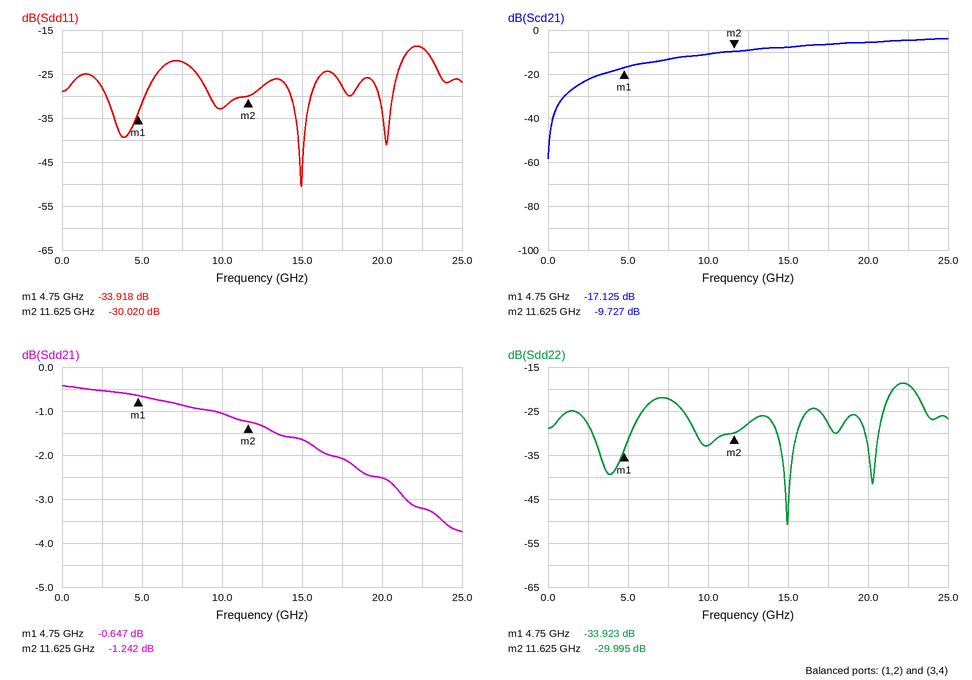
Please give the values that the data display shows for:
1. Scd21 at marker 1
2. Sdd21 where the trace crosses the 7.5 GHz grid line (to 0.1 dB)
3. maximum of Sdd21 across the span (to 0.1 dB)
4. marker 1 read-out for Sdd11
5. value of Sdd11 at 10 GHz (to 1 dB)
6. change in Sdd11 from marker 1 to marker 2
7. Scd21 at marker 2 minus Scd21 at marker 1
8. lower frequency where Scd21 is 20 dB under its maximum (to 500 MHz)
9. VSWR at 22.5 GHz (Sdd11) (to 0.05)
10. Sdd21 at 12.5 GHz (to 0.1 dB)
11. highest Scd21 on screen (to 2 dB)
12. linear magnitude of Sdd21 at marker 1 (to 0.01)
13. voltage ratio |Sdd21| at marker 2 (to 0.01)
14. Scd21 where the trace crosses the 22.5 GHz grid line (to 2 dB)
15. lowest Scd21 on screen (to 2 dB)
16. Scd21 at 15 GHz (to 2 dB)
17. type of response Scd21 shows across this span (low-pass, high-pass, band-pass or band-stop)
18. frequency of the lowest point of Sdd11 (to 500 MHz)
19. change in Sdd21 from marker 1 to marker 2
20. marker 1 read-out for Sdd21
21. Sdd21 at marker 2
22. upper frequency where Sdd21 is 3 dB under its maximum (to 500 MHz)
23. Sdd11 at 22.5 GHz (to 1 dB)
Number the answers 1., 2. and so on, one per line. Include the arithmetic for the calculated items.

1. -17.125 dB
2. -0.9 dB
3. -0.4 dB
4. -33.918 dB
5. -33 dB
6. -30.02 − (-33.918) = 3.898 dB
7. -9.727 − (-17.125) = 7.398 dB
8. 2.0 GHz
9. |Γ| = 10^(-19/20) = 0.1122; VSWR = (1 + 0.1122)/(1 − 0.1122) ≈ 1.25
10. -1.3 dB
11. -4 dB
12. 10^(-0.647/20) ≈ 0.93
13. 10^(-1.242/20) ≈ 0.87
14. -4 dB
15. -58 dB
16. -8 dB
17. high-pass
18. 15.0 GHz
19. -1.242 − (-0.647) = -0.595 dB
20. -0.647 dB
21. -1.242 dB
22. 23.5 GHz
23. -19 dB
